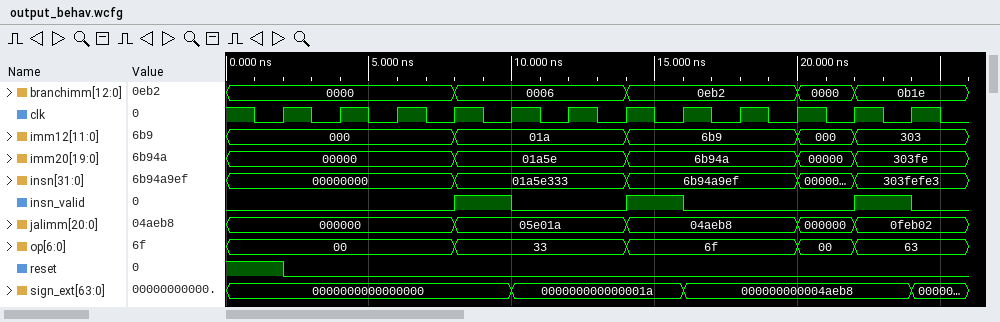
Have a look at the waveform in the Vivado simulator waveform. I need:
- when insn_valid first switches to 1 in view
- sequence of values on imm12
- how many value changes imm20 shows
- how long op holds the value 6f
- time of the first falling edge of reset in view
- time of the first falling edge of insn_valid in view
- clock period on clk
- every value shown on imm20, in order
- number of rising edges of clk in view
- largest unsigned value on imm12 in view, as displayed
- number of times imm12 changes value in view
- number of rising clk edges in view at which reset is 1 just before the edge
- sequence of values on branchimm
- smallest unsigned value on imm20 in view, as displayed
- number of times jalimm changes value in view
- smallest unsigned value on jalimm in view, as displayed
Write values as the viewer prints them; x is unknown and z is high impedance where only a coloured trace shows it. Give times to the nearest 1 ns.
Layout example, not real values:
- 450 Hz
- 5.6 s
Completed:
- 8 ns
- 000, 01a, 6b9, 000, 303
- 4
- 6 ns
- 2 ns
- 10 ns
- 2 ns
- 00000, 01a5e, 6b94a, 00000, 303fe
- 12
- 6b9
- 4
- 1
- 0000, 0006, 0eb2, 0000, 0b1e
- 00000
- 4
- 000000
